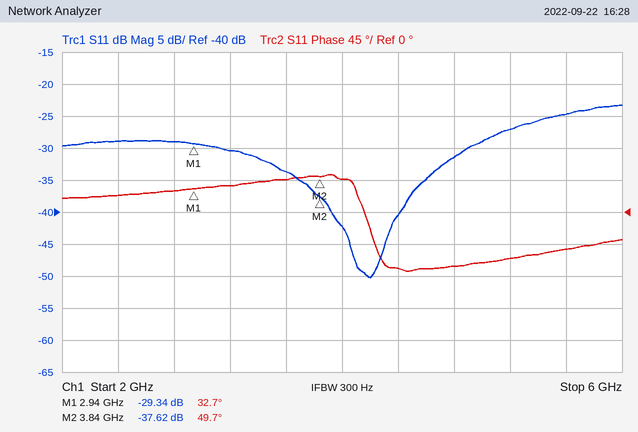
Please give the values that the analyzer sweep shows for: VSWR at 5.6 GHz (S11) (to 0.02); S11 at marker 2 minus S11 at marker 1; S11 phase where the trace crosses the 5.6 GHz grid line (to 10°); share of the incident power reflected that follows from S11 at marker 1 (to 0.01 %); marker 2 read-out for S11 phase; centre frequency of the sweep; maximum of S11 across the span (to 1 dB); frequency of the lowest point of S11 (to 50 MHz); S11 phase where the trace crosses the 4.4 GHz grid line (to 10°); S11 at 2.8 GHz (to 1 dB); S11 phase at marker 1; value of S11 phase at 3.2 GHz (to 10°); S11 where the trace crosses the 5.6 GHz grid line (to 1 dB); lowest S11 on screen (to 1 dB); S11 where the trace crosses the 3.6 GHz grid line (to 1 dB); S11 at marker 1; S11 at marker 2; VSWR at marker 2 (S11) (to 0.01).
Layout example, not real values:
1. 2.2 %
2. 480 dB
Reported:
1. 1.12
2. -8.28 dB
3. -50°
4. 0.12 %
5. 49.7°
6. 4 GHz
7. -23 dB
8. 4.20 GHz
9. -80°
10. -29 dB
11. 32.7°
12. 40°
13. -25 dB
14. -50 dB
15. -34 dB
16. -29.34 dB
17. -37.62 dB
18. 1.03
